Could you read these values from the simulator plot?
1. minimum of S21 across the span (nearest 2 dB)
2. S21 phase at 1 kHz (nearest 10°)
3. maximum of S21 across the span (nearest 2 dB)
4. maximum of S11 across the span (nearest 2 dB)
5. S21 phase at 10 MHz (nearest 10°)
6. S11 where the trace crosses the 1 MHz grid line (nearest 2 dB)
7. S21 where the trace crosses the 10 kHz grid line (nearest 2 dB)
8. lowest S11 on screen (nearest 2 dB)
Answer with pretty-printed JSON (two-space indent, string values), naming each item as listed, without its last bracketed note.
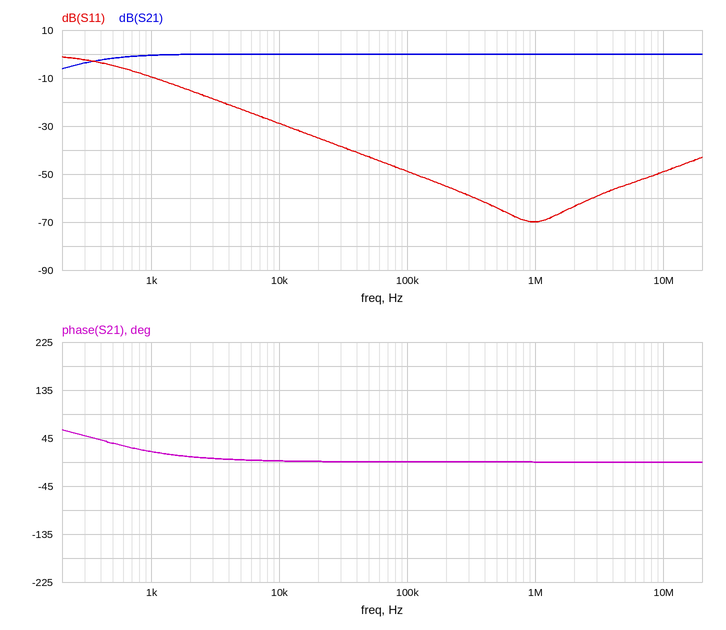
{
  "minimum of S21 across the span": "-6 dB",
  "S21 phase at 1 kHz": "20°",
  "maximum of S21 across the span": "0 dB",
  "maximum of S11 across the span": "-2 dB",
  "S21 phase at 10 MHz": "0°",
  "S11 where the trace crosses the 1 MHz grid line": "-70 dB",
  "S21 where the trace crosses the 10 kHz grid line": "0 dB",
  "lowest S11 on screen": "-70 dB"
}
